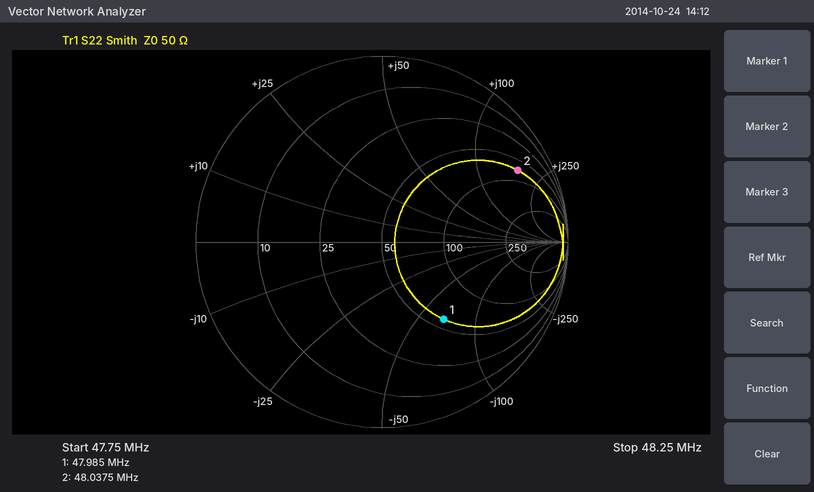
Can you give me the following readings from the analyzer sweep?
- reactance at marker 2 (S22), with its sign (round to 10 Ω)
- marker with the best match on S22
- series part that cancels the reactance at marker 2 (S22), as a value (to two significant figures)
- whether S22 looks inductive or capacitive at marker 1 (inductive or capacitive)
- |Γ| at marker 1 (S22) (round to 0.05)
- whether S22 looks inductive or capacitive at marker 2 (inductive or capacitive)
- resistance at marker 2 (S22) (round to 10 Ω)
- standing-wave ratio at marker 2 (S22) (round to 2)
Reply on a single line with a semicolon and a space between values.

+170 Ω; marker 1; 19 pF; capacitive; 0.55; inductive; 70 Ω; 10
